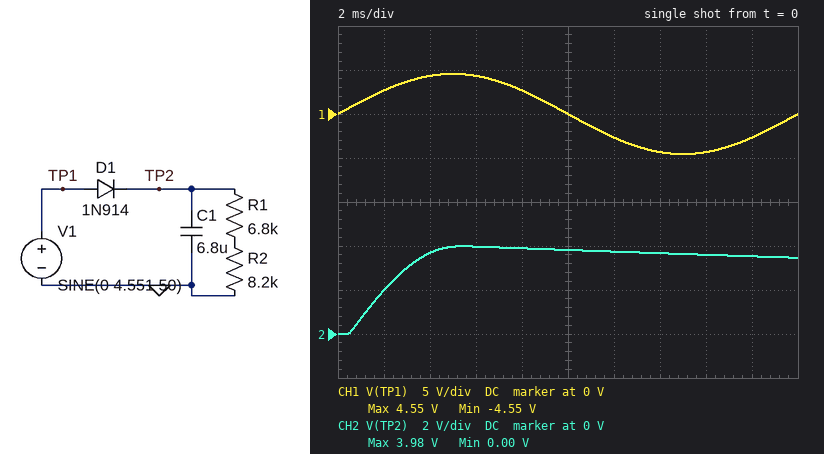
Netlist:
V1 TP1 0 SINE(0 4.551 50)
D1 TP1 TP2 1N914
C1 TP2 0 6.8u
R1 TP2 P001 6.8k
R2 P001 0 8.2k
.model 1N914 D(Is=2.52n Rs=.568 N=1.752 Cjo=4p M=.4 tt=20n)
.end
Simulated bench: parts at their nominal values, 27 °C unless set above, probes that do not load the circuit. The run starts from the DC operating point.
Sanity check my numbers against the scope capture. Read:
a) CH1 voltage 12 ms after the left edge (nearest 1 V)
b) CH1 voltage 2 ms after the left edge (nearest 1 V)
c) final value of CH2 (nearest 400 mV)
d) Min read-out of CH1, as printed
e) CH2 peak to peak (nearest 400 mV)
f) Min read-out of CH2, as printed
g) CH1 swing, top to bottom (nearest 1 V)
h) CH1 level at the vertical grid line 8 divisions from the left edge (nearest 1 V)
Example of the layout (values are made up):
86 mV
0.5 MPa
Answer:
-3 V
3 V
3.6 V
-4.55 V
4.0 V
0.00 V
9 V
-4 V
